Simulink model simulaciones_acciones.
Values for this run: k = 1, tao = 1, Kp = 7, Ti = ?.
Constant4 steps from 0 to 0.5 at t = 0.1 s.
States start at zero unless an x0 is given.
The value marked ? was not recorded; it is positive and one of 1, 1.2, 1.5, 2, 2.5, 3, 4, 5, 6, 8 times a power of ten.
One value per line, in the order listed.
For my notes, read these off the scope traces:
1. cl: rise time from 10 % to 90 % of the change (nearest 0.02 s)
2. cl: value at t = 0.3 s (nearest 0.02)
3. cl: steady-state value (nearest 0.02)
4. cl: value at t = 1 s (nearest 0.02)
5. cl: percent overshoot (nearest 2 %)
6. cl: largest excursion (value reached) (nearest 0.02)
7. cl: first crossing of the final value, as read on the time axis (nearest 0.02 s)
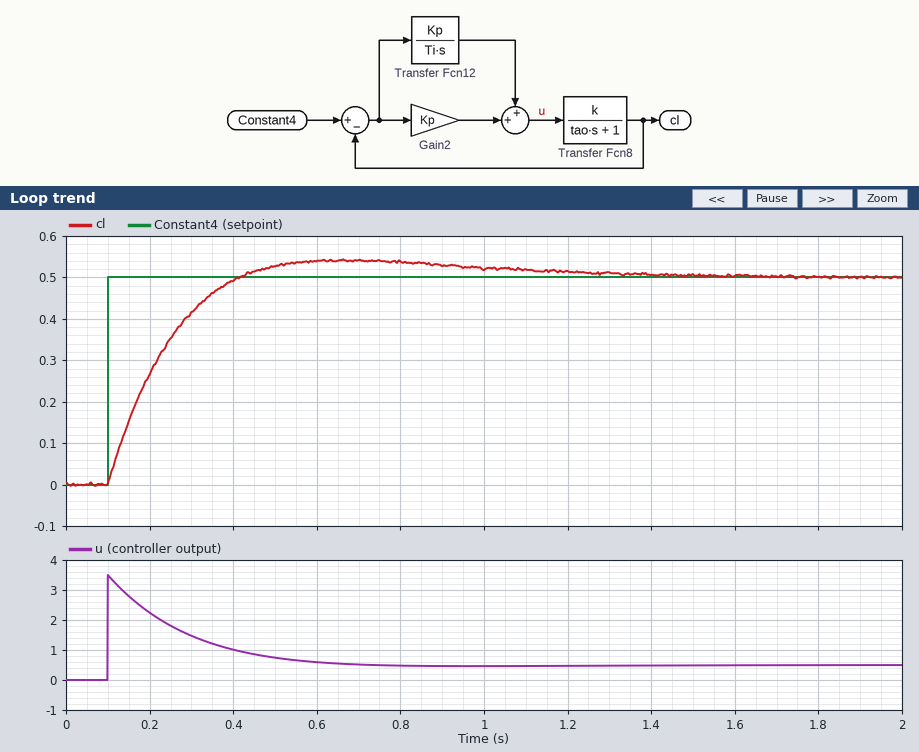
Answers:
0.22 s
0.42
0.50
0.52
8 %
0.54
0.42 s
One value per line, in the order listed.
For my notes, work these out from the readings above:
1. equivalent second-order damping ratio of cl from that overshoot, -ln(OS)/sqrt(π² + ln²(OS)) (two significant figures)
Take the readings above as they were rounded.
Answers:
0.63
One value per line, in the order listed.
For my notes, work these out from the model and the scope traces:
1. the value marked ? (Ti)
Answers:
0.4
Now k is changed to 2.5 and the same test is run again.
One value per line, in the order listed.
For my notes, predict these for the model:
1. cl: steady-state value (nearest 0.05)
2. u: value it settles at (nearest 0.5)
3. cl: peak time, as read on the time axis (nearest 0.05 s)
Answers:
0.50
0.0
0.40 s
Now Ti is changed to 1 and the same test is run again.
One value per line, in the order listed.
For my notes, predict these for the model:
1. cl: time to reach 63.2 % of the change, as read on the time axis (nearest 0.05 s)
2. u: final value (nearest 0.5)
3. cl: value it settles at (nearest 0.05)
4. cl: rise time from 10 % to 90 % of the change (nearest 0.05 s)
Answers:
0.25 s
0.5
0.50
0.30 s
